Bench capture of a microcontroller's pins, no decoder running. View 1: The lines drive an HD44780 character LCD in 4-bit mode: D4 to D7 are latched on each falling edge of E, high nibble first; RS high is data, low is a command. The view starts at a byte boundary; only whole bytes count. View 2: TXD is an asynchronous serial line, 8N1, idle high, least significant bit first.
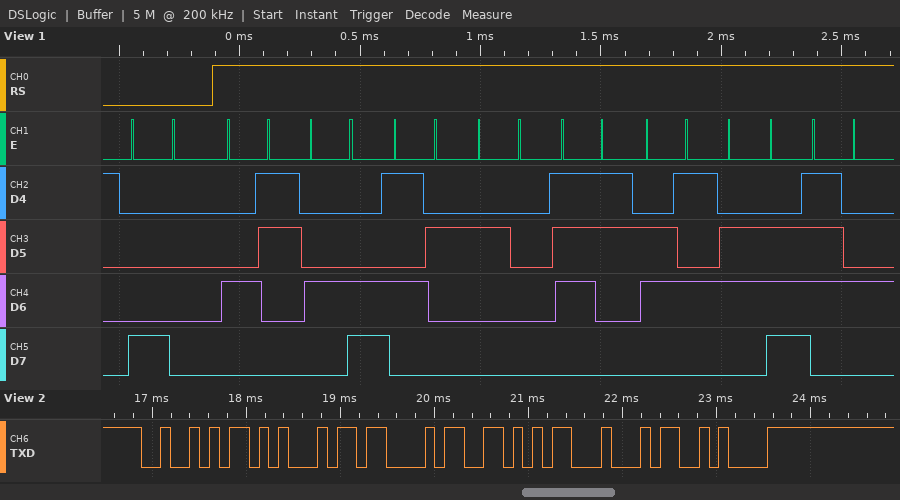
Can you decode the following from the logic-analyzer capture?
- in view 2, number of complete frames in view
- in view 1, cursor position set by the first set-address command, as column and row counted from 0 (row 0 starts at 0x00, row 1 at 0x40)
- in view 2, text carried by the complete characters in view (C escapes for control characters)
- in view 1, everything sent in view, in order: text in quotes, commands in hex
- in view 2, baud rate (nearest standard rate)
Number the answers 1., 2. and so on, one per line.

1. 6
2. column 0, row 0
3. "RECVD\n"
4. 0x80 "CLR sent"
5. 9600 baud
